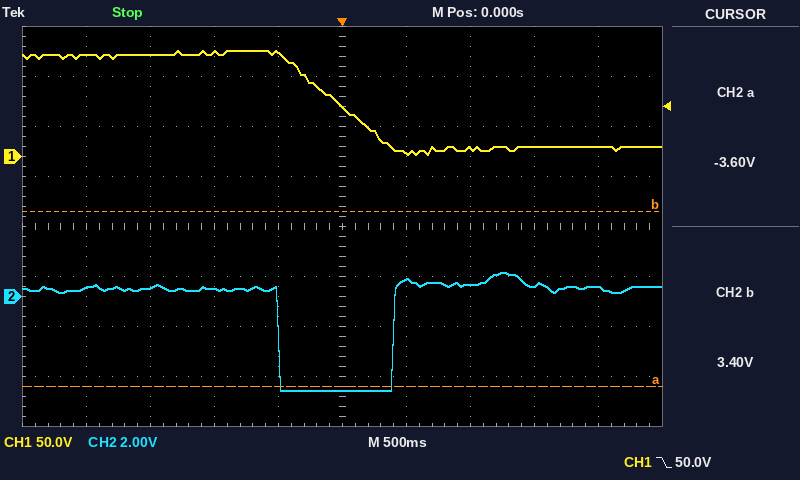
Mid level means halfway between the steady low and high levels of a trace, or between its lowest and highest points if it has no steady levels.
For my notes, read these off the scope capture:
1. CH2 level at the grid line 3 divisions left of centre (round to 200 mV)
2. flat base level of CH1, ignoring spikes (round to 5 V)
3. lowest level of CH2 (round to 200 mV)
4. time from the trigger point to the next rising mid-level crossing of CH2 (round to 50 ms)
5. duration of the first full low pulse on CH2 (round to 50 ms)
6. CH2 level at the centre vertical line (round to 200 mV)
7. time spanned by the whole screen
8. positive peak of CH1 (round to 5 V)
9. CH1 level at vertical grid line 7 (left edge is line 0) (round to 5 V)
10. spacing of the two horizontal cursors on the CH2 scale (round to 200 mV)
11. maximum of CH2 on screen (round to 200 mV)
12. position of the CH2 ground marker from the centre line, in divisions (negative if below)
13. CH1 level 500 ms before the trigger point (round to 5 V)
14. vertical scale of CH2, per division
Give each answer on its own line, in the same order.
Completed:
400 mV
10 V
-3.8 V
400 ms
900 ms
-3.8 V
5 s
105 V
10 V
7.0 V
1.0 V
-1.4 div
105 V
2 V
